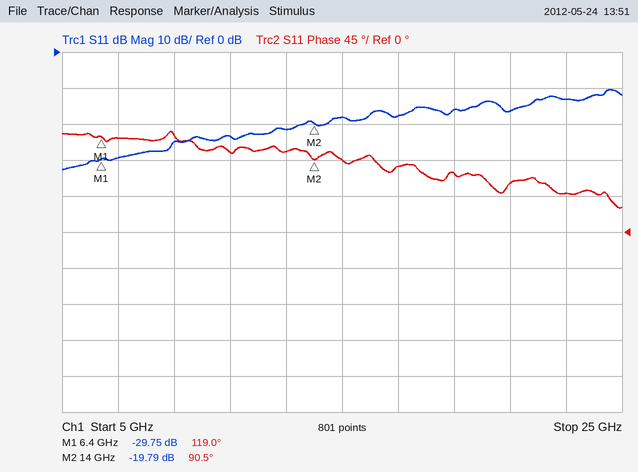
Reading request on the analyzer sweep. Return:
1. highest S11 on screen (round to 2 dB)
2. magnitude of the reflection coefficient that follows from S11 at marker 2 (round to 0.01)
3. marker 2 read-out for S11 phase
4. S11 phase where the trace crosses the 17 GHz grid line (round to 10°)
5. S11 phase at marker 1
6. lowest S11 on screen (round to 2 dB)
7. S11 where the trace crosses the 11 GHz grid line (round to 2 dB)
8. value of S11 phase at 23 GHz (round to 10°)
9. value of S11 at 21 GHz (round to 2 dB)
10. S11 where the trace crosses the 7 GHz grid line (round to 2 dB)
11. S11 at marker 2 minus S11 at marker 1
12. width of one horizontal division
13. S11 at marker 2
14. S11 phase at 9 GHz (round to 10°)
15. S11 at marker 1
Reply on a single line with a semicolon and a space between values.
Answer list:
-10 dB; 0.10; 90.5°; 80°; 119.0°; -32 dB; -24 dB; 50°; -16 dB; -30 dB; 9.96 dB; 2 GHz; -19.79 dB; 120°; -29.75 dB
